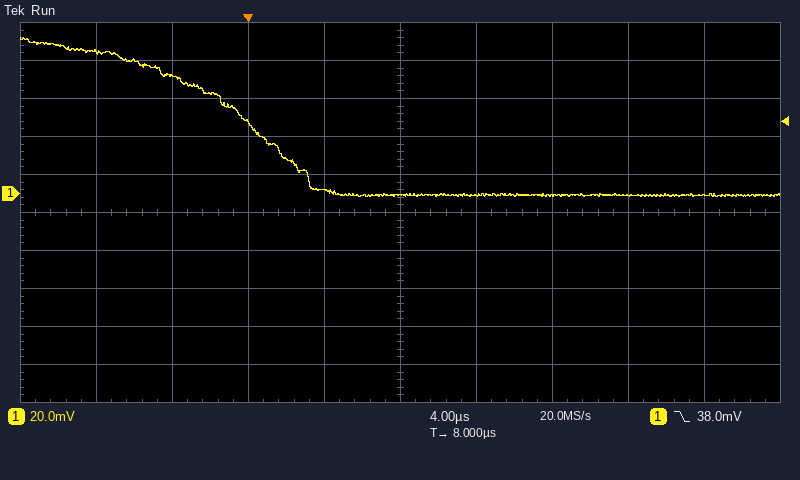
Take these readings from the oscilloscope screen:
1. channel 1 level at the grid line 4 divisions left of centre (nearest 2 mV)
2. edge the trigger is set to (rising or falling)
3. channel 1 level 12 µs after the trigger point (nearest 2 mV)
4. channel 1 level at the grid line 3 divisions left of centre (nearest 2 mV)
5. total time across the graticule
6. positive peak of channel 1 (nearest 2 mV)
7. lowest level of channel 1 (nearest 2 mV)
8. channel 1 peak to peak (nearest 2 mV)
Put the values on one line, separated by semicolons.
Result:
74 mV; falling; 0 mV; 62 mV; 40 µs; 82 mV; -2 mV; 84 mV
